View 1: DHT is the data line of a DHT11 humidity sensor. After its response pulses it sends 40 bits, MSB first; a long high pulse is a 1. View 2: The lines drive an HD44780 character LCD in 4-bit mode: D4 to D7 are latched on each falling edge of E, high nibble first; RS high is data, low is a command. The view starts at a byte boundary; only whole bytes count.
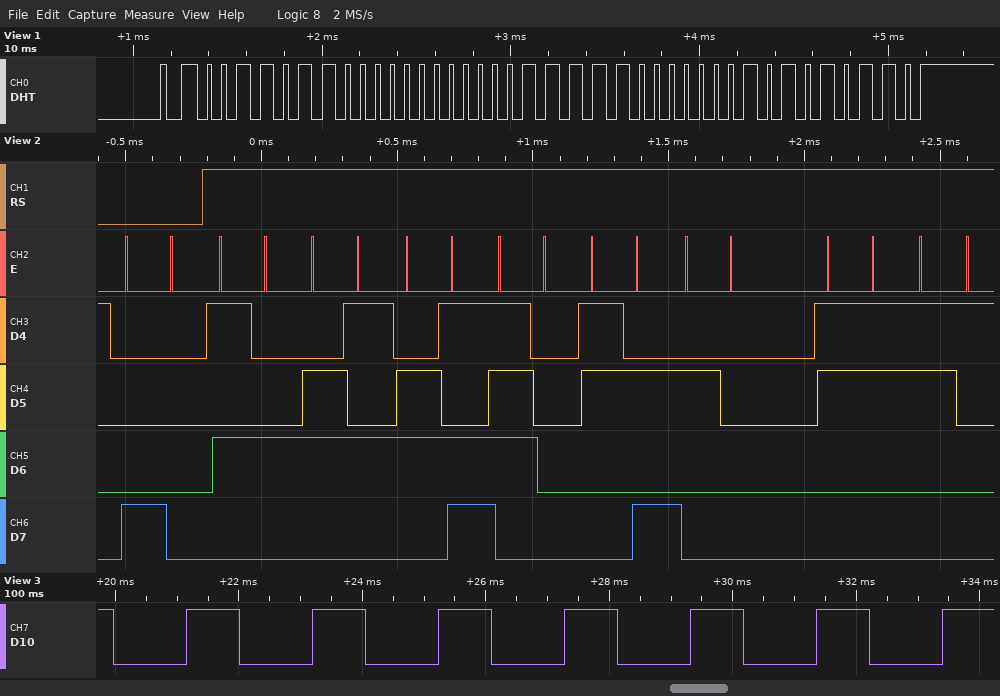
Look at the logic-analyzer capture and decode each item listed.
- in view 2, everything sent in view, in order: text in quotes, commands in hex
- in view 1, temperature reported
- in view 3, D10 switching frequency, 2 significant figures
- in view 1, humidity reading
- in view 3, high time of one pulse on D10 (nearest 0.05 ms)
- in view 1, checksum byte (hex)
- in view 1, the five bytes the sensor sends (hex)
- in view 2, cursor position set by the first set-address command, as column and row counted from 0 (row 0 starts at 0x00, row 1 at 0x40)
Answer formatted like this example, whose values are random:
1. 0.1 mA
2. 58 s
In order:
1. 0x80 "Temp: 31"
2. 31.1 °C
3. 490 Hz
4. 54 %
5. 0.85 ms
6. 0x56
7. 36 00 1F 01 56
8. column 0, row 0
